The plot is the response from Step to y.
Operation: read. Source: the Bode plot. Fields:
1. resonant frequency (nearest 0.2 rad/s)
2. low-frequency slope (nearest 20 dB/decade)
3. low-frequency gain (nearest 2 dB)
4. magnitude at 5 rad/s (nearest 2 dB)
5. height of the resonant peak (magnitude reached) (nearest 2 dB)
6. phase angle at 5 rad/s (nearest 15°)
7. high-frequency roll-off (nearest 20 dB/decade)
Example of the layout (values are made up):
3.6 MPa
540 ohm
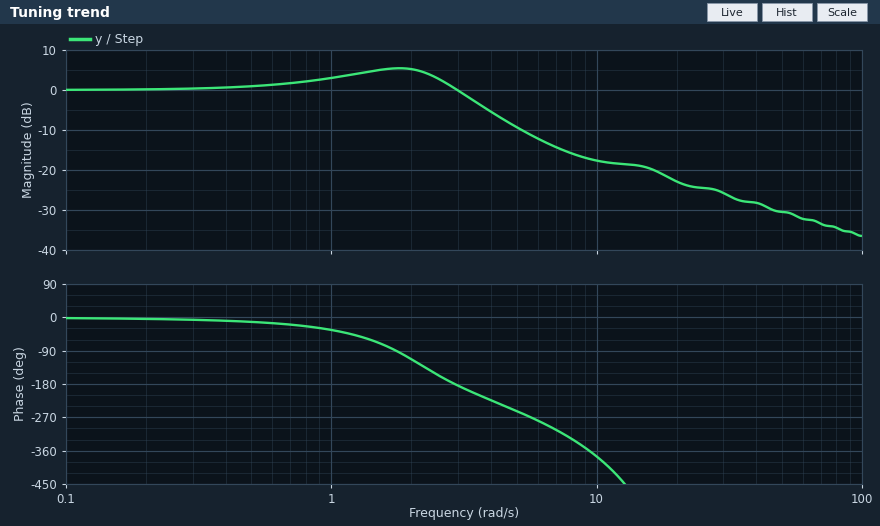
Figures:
1.8 rad/s
0 dB/decade
0 dB
-10 dB
6 dB
-255°
-20 dB/decade
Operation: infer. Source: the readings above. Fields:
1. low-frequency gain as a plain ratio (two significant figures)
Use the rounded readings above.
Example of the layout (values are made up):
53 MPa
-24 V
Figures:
1.0
